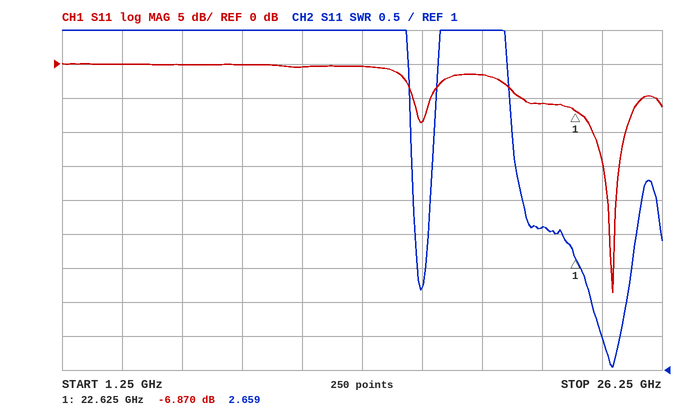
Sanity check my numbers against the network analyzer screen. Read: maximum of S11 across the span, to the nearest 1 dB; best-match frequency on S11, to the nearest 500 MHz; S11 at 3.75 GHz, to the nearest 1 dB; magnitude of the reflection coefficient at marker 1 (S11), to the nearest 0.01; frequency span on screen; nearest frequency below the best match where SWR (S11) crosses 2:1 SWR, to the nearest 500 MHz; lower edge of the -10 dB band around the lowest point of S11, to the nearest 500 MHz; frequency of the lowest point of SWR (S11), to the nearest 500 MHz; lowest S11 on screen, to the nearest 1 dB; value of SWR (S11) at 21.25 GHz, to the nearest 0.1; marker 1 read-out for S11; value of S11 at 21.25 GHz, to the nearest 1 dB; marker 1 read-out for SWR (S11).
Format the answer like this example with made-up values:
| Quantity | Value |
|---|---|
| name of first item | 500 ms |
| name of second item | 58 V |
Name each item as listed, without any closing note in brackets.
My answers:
| Quantity | Value |
|---|---|
| maximum of S11 across the span, to the nearest 1 dB | 0 dB |
| best-match frequency on S11, to the nearest 500 MHz | 24.0 GHz |
| S11 at 3.75 GHz, to the nearest 1 dB | 0 dB |
| magnitude of the reflection coefficient at marker 1 (S11), to the nearest 0.01 | 0.45 |
| frequency span on screen | 25 GHz |
| nearest frequency below the best match where SWR (S11) crosses 2:1 SWR, to the nearest 500 MHz | 23.5 GHz |
| lower edge of the -10 dB band around the lowest point of S11, to the nearest 500 MHz | 23.5 GHz |
| frequency of the lowest point of SWR (S11), to the nearest 500 MHz | 24.0 GHz |
| lowest S11 on screen, to the nearest 1 dB | -34 dB |
| value of SWR (S11) at 21.25 GHz, to the nearest 0.1 | 3.1 |
| marker 1 read-out for S11 | -6.870 dB |
| value of S11 at 21.25 GHz, to the nearest 1 dB | -6 dB |
| marker 1 read-out for SWR | 2.659 |
